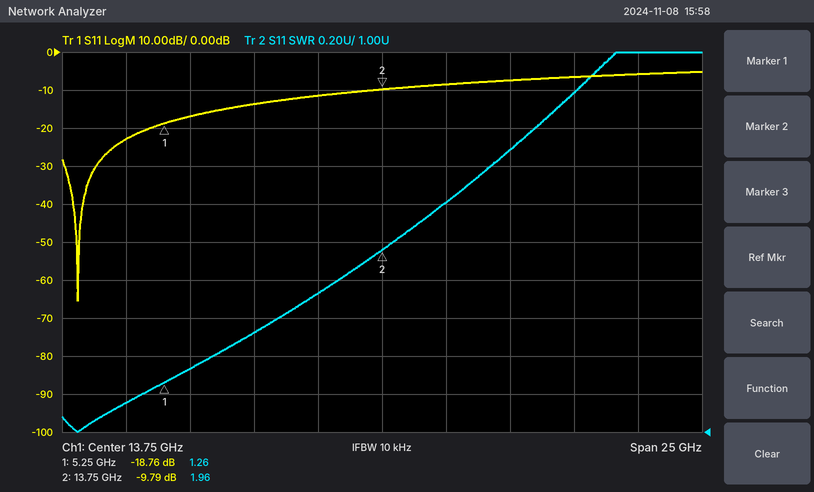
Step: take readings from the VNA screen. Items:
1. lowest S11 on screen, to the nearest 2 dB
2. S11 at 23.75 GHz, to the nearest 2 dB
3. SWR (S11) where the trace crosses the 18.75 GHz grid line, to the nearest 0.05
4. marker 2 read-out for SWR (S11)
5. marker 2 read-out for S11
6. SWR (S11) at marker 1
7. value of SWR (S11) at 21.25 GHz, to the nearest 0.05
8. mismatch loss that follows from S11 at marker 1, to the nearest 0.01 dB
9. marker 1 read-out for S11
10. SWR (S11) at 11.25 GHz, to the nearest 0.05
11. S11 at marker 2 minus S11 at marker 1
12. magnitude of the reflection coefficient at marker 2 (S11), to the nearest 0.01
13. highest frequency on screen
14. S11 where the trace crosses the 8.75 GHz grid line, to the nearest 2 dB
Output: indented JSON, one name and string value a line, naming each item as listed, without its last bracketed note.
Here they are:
{
  "lowest S11 on screen, to the nearest 2 dB": "-66 dB",
  "S11 at 23.75 GHz, to the nearest 2 dB": "-6 dB",
  "SWR (S11) where the trace crosses the 18.75 GHz grid line, to the nearest 0.05": "2.50",
  "marker 2 read-out for SWR": "1.96",
  "marker 2 read-out for S11": "-9.79 dB",
  "SWR (S11) at marker 1": "1.26",
  "value of SWR (S11) at 21.25 GHz, to the nearest 0.05": "2.80",
  "mismatch loss that follows from S11 at marker 1, to the nearest 0.01 dB": "0.06 dB",
  "marker 1 read-out for S11": "-18.76 dB",
  "SWR (S11) at 11.25 GHz, to the nearest 0.05": "1.75",
  "S11 at marker 2 minus S11 at marker 1": "8.97 dB",
  "magnitude of the reflection coefficient at marker 2 (S11), to the nearest 0.01": "0.32",
  "highest frequency on screen": "26.25 GHz",
  "S11 where the trace crosses the 8.75 GHz grid line, to the nearest 2 dB": "-14 dB"
}
